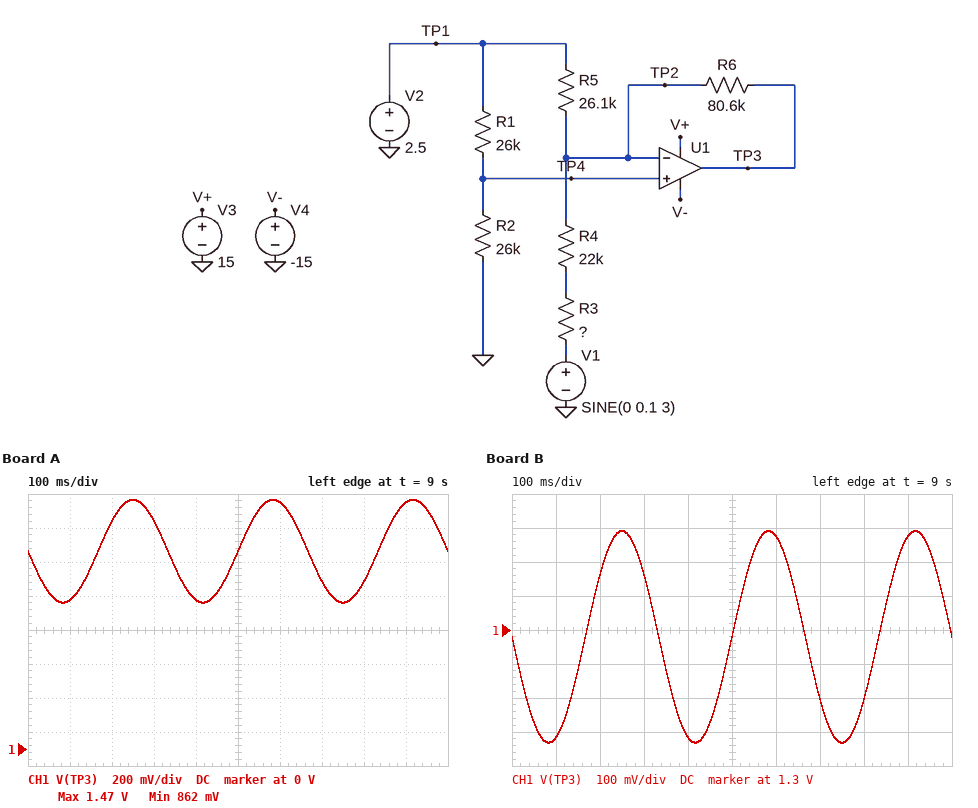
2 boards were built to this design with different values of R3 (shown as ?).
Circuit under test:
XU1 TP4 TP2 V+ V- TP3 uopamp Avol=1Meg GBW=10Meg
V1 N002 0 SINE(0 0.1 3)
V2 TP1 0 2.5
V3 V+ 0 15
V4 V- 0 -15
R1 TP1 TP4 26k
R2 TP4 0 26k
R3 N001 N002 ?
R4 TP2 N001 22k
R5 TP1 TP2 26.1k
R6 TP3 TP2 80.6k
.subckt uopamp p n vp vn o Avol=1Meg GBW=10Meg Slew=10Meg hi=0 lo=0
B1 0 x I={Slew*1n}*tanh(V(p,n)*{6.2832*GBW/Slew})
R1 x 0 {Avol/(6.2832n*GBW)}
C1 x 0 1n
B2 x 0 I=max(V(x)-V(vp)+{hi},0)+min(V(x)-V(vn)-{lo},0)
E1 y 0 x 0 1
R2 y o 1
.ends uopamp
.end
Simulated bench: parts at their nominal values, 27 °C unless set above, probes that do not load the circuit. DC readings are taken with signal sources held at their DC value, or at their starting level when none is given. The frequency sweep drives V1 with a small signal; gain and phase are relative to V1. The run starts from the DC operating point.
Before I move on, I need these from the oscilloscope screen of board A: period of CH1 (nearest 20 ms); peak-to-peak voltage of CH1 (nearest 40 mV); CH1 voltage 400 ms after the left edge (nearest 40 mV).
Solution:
340 ms
600 mV
880 mV
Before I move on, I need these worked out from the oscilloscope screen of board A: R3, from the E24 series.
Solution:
4.7 kΩ
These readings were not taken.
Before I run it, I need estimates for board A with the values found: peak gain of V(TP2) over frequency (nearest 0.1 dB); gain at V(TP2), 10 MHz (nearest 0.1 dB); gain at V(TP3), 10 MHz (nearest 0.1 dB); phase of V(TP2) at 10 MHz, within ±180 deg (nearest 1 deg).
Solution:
-7.4 dB
-7.5 dB
-7.5 dB
8 deg
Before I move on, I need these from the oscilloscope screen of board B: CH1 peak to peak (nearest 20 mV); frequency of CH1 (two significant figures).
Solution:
620 mV
3.0 Hz
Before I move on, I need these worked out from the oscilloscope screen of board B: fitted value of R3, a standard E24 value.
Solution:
3.9 kΩ
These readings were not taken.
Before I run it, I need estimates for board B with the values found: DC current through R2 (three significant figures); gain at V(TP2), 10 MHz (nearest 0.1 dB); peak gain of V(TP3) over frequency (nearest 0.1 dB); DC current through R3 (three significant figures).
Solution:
48.1 µA
-7.4 dB
9.9 dB
48.3 µA
